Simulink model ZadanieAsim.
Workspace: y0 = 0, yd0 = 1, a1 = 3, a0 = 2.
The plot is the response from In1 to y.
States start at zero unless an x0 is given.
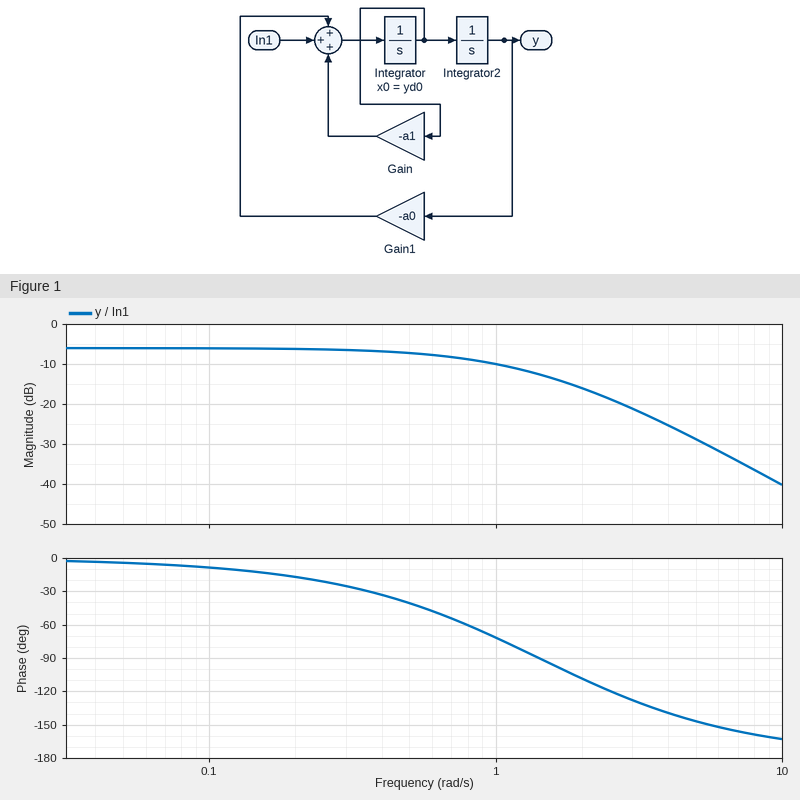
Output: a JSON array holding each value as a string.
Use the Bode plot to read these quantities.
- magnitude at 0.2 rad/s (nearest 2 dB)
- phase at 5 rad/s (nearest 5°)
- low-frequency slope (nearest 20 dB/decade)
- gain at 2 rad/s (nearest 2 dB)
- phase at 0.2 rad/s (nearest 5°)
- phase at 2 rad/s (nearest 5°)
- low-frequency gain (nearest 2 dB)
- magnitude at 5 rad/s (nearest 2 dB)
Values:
["-6 dB", "-145°", "0 dB/decade", "-16 dB", "-15°", "-110°", "-6 dB", "-28 dB"]
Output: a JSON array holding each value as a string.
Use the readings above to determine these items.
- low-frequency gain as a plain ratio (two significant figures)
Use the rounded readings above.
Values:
["0.50"]
